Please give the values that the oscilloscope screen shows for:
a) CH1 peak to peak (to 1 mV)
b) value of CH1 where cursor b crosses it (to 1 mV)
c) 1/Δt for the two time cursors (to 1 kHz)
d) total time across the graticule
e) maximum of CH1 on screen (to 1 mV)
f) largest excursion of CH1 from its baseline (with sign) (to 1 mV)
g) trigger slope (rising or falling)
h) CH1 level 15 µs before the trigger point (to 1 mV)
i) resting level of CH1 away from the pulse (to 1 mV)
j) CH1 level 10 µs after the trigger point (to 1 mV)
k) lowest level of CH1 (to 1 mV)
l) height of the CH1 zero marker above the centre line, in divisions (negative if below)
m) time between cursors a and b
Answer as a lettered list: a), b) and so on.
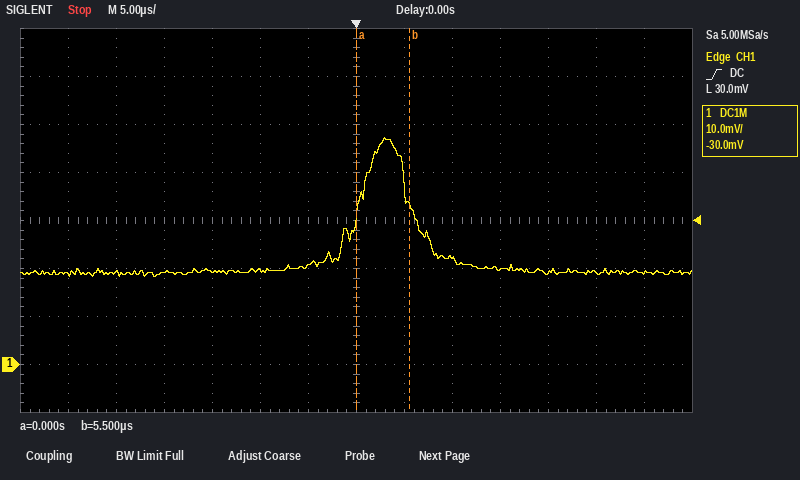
a) 29 mV
b) 33 mV
c) 182 kHz
d) 70 µs
e) 47 mV
f) +28 mV
g) rising
h) 19 mV
i) 19 mV
j) 22 mV
k) 18 mV
l) -3.0 div
m) 5.5 µs
